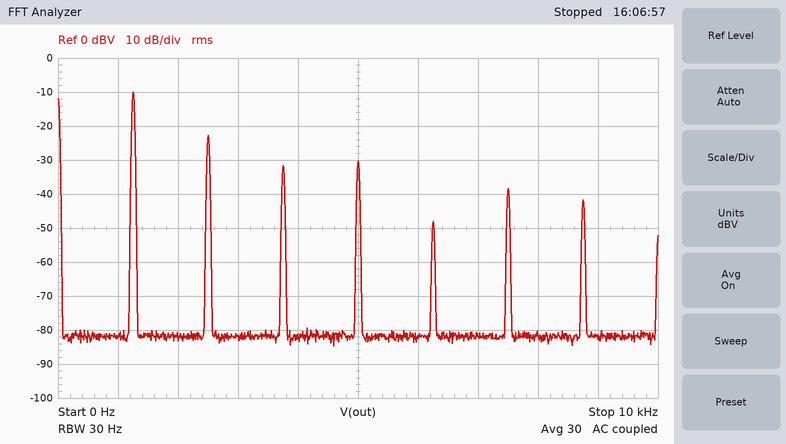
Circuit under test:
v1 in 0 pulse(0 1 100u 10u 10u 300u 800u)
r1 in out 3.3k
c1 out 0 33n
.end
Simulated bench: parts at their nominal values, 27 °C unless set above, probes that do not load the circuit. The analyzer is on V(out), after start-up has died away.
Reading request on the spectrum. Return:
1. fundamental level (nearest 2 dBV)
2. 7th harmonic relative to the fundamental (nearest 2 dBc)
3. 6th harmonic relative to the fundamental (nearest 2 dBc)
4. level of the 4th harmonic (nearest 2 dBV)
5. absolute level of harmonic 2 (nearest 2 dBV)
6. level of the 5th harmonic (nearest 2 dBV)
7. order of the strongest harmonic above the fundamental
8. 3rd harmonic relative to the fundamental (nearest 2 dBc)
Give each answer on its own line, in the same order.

-10 dBV
-32 dBc
-28 dBc
-30 dBV
-22 dBV
-48 dBV
2
-22 dBc
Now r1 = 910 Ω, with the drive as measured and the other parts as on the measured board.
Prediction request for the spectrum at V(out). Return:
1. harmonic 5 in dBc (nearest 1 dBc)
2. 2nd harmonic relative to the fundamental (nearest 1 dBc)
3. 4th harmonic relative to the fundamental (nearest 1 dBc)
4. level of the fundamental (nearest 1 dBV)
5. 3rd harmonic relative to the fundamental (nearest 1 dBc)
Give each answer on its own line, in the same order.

-31 dBc
-10 dBc
-14 dBc
-8 dBV
-17 dBc
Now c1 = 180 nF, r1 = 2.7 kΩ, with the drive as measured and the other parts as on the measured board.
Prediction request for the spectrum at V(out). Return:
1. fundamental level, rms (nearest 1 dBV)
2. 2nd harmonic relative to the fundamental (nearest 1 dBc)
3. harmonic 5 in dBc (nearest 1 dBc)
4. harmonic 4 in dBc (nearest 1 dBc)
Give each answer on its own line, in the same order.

-19 dBV
-15 dBc
-41 dBc
-23 dBc
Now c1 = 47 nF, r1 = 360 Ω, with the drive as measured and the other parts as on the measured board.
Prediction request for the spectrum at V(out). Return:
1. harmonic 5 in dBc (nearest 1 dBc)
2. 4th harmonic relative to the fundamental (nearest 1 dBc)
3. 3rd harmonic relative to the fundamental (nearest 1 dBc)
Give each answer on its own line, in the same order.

-29 dBc
-13 dBc
-16 dBc
